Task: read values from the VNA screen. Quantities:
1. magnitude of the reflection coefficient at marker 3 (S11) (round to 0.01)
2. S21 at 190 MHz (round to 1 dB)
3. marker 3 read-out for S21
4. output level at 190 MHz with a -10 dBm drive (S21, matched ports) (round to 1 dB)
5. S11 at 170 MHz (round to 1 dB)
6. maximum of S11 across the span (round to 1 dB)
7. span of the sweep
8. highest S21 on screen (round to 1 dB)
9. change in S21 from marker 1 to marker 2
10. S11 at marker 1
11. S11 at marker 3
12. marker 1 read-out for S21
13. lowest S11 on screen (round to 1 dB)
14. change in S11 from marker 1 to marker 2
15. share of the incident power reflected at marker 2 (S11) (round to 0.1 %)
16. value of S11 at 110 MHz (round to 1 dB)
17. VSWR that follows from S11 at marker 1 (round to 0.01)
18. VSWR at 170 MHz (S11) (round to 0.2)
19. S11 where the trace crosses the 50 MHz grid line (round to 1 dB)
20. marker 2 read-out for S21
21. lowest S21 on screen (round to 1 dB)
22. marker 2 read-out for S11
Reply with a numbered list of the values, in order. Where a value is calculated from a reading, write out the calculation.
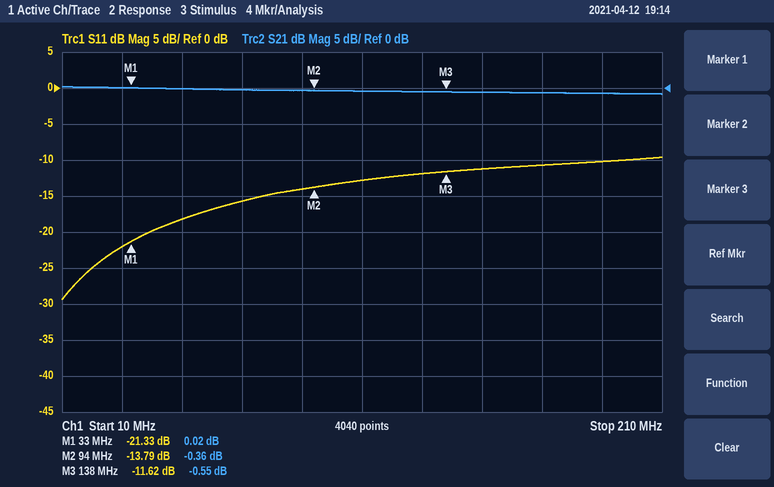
1. 10^(-11.62/20) ≈ 0.26
2. -1 dB
3. -0.55 dB
4. -10 dBm + (-1 dB) = -11 dBm
5. -11 dB
6. -10 dB
7. 200 MHz
8. 0 dB
9. -0.36 − (0.02) = -0.38 dB
10. -21.33 dB
11. -11.62 dB
12. 0.02 dB
13. -29 dB
14. -13.79 − (-21.33) = 7.54 dB
15. 10^(-13.79/10) ≈ 4.2 %
16. -13 dB
17. (1 + 0.0858)/(1 − 0.0858) ≈ 1.19
18. |Γ| = 10^(-11/20) = 0.2818; VSWR = (1 + 0.2818)/(1 − 0.2818) ≈ 1.8
19. -18 dB
20. -0.36 dB
21. -1 dB
22. -13.79 dB
